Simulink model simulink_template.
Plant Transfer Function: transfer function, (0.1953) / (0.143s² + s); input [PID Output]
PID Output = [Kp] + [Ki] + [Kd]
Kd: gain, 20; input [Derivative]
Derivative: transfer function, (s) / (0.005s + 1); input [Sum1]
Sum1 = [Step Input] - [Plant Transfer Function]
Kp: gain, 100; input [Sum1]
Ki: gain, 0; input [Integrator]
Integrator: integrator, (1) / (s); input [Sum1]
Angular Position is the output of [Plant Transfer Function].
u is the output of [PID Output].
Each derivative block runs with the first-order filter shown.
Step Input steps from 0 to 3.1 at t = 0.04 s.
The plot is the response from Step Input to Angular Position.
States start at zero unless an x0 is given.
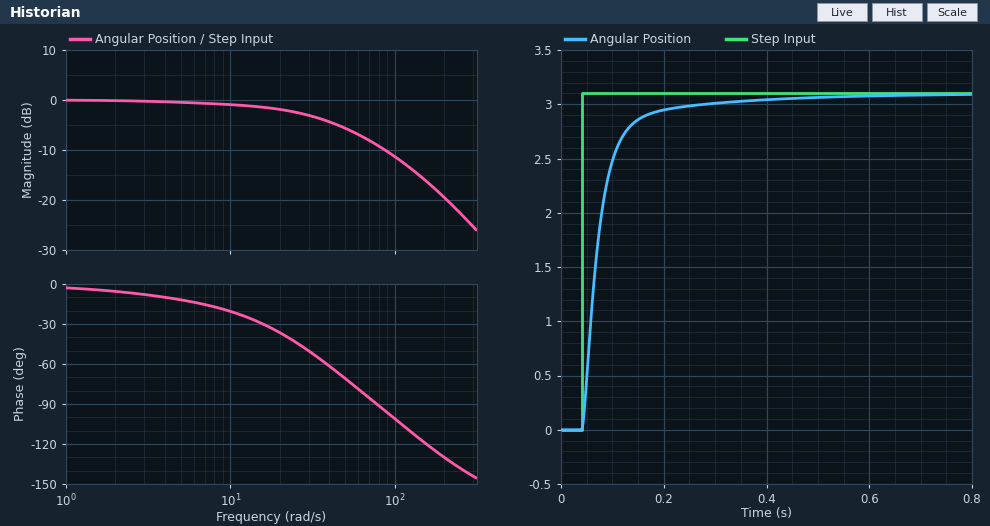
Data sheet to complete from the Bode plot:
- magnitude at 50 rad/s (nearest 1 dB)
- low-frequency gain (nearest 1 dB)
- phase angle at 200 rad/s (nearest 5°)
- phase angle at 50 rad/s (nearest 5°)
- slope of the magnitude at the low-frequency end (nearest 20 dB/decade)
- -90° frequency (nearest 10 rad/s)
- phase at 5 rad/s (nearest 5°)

-6 dB
0 dB
-130°
-70°
0 dB/decade
80 rad/s
-10°
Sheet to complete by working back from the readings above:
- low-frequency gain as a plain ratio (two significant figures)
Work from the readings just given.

1.0
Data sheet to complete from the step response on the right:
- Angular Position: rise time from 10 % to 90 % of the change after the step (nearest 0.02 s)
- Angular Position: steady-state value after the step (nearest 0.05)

0.08 s
3.10
